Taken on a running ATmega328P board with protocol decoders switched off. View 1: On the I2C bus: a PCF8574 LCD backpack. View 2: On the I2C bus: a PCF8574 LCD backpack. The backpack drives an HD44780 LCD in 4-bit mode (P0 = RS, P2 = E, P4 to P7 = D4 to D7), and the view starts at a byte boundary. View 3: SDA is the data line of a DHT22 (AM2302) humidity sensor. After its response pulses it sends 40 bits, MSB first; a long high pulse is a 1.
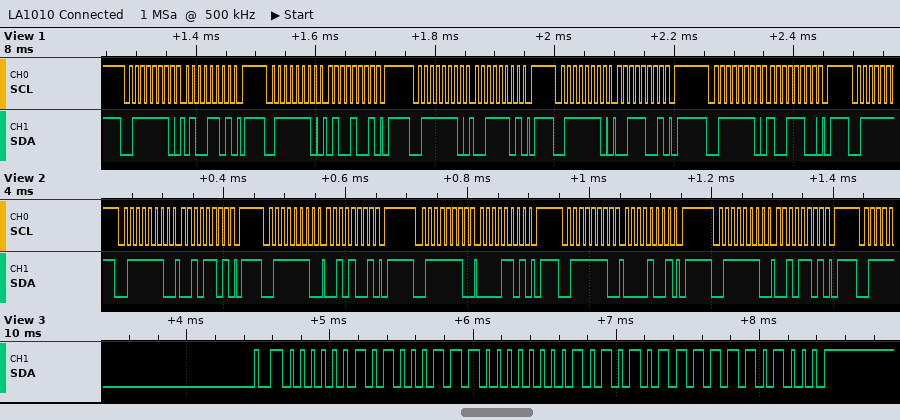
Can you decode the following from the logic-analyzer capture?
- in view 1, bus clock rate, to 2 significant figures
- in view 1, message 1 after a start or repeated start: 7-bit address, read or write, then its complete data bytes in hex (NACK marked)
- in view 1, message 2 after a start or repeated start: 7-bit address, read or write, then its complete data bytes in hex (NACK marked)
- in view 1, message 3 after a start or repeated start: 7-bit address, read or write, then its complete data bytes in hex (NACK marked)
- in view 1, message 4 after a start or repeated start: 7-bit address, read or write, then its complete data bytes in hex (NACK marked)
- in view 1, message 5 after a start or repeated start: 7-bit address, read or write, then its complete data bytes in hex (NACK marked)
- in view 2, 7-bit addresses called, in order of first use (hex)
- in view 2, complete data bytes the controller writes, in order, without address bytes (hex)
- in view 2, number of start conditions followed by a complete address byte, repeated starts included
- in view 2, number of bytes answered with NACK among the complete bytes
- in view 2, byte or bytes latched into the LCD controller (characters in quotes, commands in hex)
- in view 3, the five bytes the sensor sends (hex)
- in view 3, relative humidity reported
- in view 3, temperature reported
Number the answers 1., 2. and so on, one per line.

1. 100 kHz
2. 0x3F write: 4D
3. 0x3F write: 49
4. 0x3F write: 3D
5. 0x3F write: 39
6. 0x3F write: 9C
7. 0x3F
8. 2D 29 0D 09 2D
9. 5
10. 0
11. ' '
12. 02 8E 01 57 E8
13. 65.4 %
14. 34.3 °C
